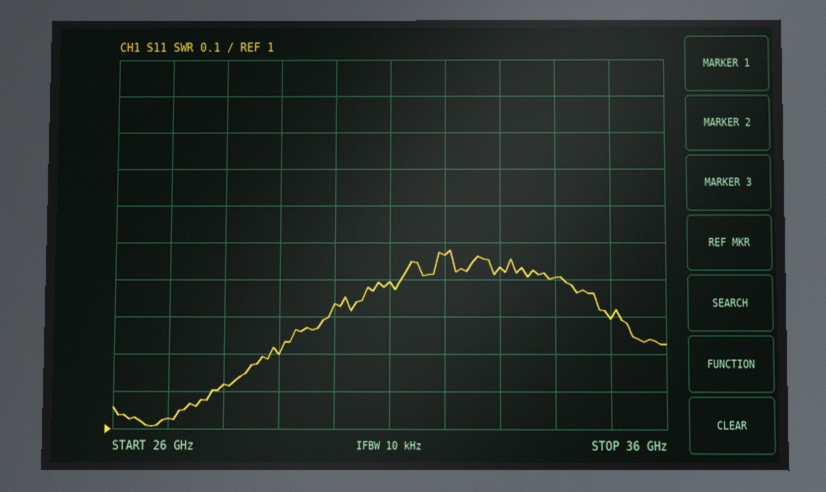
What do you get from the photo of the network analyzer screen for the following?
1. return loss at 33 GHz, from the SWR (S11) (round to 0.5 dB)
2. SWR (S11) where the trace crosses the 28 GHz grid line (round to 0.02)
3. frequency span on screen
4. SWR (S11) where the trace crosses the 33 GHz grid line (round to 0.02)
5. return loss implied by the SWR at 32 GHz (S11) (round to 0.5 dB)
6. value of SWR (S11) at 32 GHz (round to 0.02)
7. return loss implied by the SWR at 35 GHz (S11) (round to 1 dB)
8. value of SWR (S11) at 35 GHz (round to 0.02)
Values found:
15.0 dB
1.12
10 GHz
1.44
14.5 dB
1.46
18 dB
1.30
